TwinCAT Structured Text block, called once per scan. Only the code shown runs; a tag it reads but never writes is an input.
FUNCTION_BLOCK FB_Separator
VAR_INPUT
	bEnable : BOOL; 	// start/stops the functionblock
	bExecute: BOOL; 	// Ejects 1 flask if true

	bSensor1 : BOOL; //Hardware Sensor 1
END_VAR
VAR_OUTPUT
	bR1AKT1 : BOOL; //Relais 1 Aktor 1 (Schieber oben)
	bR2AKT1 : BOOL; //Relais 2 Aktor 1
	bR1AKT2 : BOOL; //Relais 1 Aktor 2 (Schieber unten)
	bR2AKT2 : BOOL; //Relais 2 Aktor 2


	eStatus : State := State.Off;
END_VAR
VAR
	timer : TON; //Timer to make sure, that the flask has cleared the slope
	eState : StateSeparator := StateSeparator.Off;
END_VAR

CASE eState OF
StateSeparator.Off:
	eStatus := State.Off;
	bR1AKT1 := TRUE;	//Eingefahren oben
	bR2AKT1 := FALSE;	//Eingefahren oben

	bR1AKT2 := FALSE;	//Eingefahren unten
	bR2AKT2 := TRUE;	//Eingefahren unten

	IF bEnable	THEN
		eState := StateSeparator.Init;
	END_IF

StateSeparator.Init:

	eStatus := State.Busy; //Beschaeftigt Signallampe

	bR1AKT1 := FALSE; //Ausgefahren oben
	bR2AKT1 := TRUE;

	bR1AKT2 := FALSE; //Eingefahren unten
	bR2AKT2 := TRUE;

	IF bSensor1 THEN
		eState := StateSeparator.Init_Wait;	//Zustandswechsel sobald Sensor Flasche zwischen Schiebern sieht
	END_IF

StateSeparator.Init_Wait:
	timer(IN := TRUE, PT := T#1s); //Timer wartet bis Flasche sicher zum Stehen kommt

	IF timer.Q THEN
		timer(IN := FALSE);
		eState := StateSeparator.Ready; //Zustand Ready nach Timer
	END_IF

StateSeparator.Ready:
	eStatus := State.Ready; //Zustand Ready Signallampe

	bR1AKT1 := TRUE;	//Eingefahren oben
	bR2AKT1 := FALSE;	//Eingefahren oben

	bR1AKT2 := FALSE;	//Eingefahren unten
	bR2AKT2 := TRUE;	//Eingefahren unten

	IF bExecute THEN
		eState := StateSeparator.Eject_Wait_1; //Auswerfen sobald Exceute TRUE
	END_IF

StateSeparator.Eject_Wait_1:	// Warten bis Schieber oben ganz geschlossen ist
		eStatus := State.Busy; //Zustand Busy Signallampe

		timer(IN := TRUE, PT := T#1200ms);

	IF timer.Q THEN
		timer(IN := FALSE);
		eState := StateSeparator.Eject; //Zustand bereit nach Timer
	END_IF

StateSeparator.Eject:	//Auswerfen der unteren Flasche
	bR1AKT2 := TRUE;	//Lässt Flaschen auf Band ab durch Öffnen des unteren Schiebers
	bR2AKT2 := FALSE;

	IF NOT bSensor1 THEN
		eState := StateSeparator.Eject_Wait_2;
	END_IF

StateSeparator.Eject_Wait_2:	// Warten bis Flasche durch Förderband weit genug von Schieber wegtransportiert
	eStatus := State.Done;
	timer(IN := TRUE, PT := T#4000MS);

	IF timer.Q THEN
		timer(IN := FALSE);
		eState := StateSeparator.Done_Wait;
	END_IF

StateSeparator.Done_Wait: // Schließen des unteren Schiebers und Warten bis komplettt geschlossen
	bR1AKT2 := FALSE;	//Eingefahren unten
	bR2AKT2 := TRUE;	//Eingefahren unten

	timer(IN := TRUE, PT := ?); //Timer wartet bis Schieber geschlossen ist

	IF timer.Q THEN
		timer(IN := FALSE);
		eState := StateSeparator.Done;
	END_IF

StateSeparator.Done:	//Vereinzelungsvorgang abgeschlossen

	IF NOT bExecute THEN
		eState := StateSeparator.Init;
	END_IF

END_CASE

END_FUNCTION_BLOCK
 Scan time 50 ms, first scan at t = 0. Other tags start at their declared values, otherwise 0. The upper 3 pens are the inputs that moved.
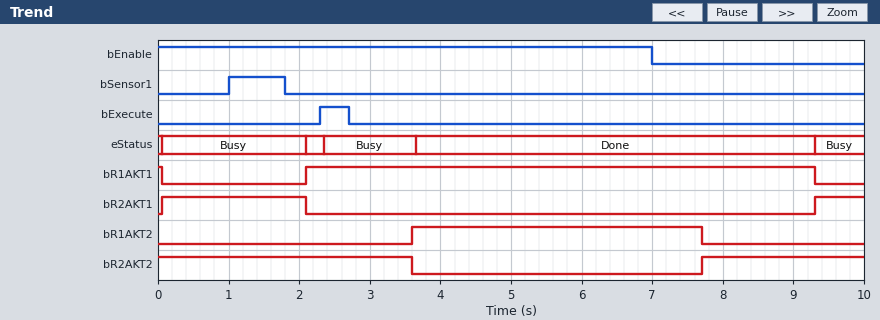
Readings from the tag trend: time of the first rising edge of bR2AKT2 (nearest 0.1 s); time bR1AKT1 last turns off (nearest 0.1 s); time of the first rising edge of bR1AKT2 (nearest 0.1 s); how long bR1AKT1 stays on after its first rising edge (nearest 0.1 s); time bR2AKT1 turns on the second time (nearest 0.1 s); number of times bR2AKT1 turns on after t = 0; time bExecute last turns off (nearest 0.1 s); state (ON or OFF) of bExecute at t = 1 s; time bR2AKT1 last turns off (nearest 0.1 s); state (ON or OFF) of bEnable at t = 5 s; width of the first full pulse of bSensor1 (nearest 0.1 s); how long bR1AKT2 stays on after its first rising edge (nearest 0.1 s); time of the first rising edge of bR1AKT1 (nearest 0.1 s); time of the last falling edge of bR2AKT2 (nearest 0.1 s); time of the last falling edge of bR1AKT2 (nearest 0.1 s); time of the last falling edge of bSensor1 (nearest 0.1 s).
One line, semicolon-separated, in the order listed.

7.7 s; 9.3 s; 3.6 s; 7.2 s; 9.3 s; 2; 2.7 s; OFF; 2.1 s; ON; 0.8 s; 4.1 s; 2.1 s; 3.6 s; 7.7 s; 1.8 s
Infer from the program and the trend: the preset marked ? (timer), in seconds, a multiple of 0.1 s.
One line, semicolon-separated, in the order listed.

1.5 s
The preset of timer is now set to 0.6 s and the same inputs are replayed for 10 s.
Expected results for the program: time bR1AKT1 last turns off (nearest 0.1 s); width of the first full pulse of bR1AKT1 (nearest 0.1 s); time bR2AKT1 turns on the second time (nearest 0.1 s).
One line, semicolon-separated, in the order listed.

8.4 s; 6.3 s; 8.4 s
